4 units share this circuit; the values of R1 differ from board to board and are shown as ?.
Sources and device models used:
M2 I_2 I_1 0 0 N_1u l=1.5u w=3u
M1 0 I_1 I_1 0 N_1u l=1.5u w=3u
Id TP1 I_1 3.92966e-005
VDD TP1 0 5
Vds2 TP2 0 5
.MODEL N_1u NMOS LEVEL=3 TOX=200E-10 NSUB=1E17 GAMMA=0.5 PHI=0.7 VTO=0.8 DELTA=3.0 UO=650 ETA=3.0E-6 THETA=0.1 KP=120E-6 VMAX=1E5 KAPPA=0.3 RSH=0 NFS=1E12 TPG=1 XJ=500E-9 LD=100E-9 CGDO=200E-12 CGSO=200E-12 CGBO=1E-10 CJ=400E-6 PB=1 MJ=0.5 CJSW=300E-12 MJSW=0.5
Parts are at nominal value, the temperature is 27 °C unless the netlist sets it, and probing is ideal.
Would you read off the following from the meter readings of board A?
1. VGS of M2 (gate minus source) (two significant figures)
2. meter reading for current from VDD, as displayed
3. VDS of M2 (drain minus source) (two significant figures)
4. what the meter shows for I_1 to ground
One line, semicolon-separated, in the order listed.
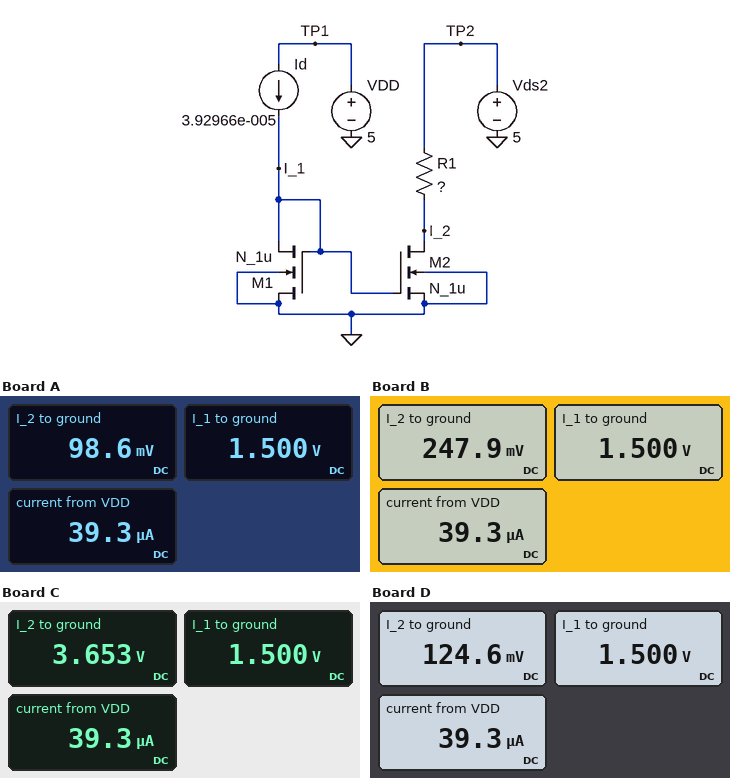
1.5 V; 39.3 µA; 99 mV; 1.500 V
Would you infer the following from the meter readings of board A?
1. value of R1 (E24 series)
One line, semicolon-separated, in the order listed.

330 kΩ
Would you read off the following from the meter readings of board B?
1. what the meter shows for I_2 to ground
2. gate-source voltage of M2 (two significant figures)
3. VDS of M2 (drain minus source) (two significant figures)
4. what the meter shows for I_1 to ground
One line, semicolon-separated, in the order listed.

247.9 mV; 1.5 V; 250 mV; 1.500 V
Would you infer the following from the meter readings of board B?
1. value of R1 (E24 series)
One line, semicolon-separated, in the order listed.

160 kΩ
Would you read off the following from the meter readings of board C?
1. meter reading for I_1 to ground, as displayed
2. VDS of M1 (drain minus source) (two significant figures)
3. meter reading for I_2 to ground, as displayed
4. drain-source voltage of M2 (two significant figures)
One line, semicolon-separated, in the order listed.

1.500 V; -1.5 V; 3.653 V; 3.7 V
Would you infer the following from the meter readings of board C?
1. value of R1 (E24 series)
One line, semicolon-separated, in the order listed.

33 kΩ
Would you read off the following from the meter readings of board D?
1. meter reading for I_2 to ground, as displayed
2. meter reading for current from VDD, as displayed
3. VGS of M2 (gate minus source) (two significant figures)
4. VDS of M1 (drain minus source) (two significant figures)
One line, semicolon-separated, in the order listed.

124.6 mV; 39.3 µA; 1.5 V; -1.5 V
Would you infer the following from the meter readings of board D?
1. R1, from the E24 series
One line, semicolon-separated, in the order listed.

270 kΩ
